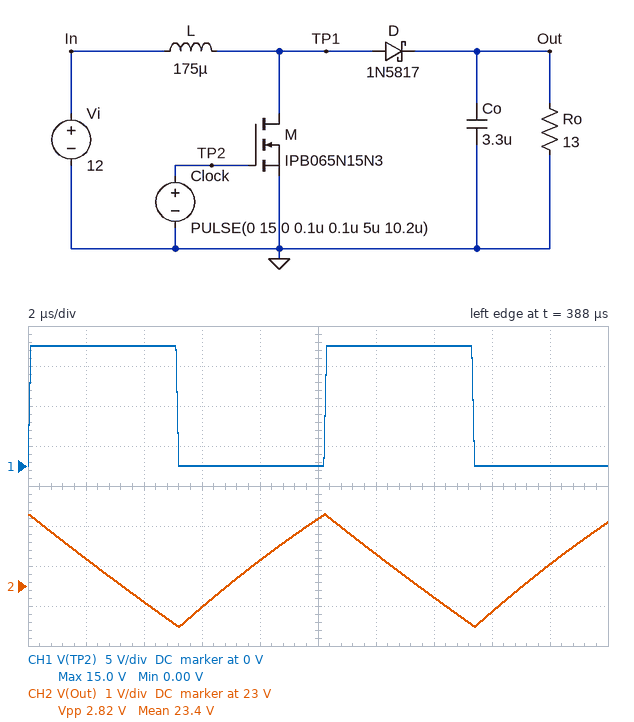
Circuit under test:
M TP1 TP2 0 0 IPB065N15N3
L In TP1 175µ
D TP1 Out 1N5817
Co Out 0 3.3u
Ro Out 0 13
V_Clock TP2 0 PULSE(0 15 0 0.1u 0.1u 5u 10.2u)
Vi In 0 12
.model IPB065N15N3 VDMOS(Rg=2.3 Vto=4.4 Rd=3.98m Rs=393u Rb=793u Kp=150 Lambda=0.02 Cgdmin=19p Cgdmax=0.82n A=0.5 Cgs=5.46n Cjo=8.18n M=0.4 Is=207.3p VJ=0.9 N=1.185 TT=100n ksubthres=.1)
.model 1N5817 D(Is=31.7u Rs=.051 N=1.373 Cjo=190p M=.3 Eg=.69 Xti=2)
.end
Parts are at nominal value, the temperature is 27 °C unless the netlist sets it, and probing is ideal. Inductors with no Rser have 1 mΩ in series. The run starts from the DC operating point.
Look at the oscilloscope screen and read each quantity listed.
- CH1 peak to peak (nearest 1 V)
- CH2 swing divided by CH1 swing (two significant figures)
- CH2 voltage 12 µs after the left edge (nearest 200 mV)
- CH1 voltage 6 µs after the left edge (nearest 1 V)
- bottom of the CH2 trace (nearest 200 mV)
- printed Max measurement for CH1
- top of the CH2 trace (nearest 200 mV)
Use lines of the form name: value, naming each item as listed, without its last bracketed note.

CH1 peak to peak: 15 V
CH2 swing divided by CH1 swing: 0.19
CH2 voltage 12 µs after the left edge: 23.8 V
CH1 voltage 6 µs after the left edge: 0 V
bottom of the CH2 trace: 22.0 V
printed Max measurement for CH1: 15.0 V
top of the CH2 trace: 24.8 V
